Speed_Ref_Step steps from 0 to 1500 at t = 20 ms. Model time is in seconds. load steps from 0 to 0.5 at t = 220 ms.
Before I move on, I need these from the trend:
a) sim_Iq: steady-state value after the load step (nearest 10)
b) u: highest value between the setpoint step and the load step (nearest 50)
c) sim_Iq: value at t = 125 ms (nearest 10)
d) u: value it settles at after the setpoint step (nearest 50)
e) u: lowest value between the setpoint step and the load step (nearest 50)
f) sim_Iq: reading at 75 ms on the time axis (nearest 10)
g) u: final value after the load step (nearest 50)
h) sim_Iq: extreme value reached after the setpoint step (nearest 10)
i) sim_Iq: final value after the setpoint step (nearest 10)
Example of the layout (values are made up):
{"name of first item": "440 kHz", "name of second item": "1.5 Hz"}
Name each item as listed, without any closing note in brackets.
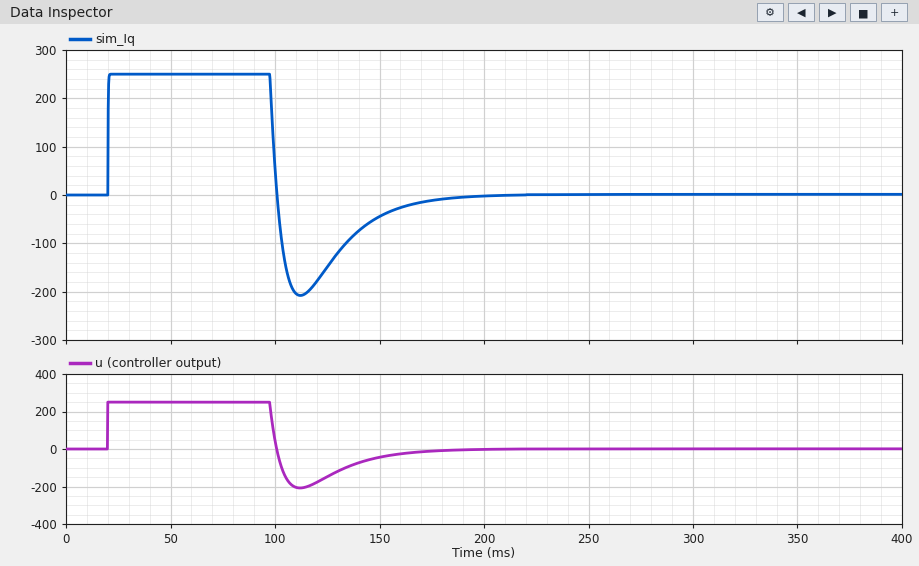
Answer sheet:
{"sim_Iq: steady-state value after the load step": "0", "u: highest value between the setpoint step and the load step": "250", "sim_Iq: value at t = 125 ms": "-150", "u: value it settles at after the setpoint step": "0", "u: lowest value between the setpoint step and the load step": "-200", "sim_Iq: reading at 75 ms on the time axis": "250", "u: final value after the load step": "0", "sim_Iq: extreme value reached after the setpoint step": "250", "sim_Iq: final value after the setpoint step": "0"}
